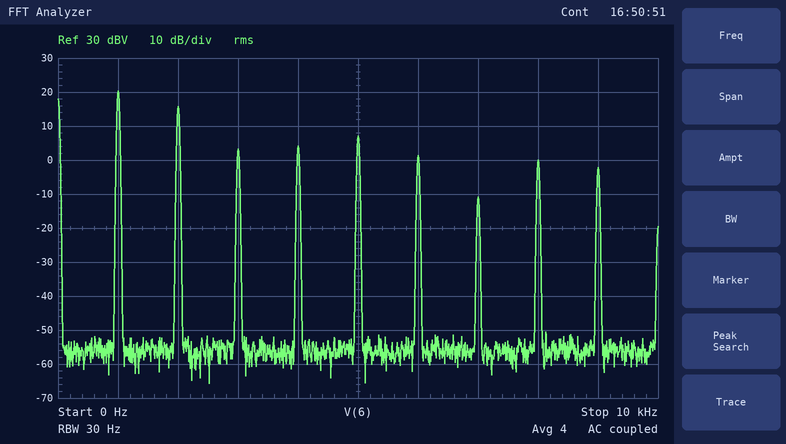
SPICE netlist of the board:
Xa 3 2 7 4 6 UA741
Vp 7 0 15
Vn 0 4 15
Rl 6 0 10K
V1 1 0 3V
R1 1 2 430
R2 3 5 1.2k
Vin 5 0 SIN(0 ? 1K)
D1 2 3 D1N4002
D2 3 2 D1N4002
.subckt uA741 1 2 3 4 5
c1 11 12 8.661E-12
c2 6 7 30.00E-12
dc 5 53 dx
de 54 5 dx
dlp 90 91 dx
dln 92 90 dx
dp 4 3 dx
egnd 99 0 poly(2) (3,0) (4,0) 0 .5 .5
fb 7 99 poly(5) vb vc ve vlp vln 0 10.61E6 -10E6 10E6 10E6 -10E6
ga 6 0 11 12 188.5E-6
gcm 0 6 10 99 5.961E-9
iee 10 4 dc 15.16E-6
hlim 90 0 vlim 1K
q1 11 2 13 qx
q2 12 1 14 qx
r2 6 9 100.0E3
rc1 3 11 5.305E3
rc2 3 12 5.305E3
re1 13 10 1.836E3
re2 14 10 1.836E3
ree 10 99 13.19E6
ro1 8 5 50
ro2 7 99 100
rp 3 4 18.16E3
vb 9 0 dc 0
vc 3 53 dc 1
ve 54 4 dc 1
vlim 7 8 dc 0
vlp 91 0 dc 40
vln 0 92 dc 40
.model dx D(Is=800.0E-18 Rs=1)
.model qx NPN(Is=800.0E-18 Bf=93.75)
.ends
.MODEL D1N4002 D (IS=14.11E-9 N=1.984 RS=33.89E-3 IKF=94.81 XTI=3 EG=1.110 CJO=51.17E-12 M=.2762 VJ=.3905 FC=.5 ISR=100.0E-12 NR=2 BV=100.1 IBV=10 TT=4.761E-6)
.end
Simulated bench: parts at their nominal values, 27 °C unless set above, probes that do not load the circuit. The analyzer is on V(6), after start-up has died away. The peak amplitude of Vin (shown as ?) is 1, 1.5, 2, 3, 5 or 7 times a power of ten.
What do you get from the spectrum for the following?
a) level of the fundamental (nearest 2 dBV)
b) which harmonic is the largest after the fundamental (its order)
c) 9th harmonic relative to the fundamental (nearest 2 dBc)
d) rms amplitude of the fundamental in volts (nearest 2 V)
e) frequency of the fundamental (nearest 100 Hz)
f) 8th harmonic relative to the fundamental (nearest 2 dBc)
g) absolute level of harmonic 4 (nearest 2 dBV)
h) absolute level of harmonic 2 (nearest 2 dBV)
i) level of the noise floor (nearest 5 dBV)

20 dBV
2
-22 dBc
10 V
1.0 kHz
-20 dBc
4 dBV
16 dBV
-55 dBV
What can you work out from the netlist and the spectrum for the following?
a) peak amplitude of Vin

5 V
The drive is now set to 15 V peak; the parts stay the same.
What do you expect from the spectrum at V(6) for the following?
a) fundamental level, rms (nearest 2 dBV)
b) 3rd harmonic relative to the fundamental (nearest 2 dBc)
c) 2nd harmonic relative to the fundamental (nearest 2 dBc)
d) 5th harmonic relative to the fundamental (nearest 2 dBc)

22 dBV
-12 dBc
-14 dBc
-20 dBc
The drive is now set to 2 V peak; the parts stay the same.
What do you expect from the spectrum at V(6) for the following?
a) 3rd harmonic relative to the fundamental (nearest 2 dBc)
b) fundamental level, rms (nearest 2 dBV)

-54 dBc
-86 dBV
